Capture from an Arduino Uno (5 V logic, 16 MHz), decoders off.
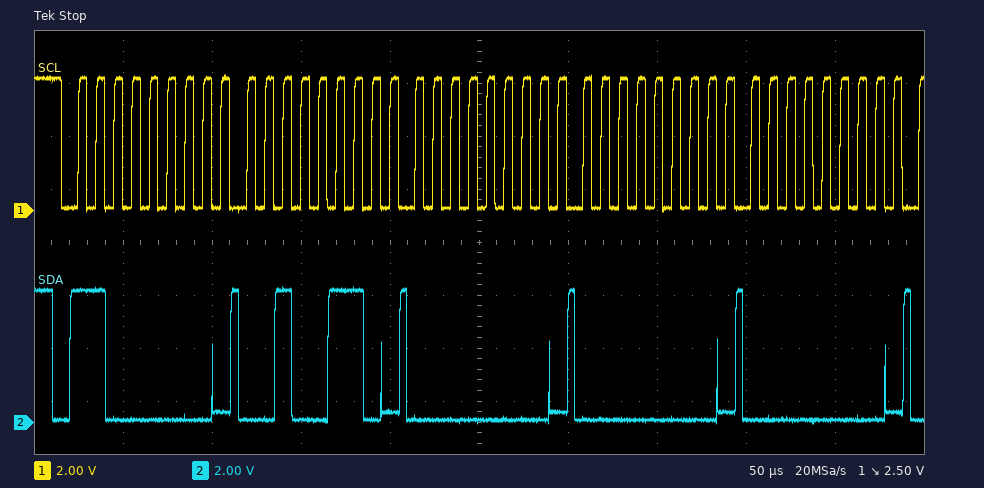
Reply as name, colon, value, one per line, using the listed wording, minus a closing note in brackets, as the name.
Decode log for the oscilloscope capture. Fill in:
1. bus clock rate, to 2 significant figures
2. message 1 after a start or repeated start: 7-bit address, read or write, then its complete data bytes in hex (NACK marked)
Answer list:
bus clock rate, to 2 significant figures: 100 kHz
message 1 after a start or repeated start: 7-bit address, read or write, then its complete data bytes in hex: 0x60 write: 26 00 00 00
